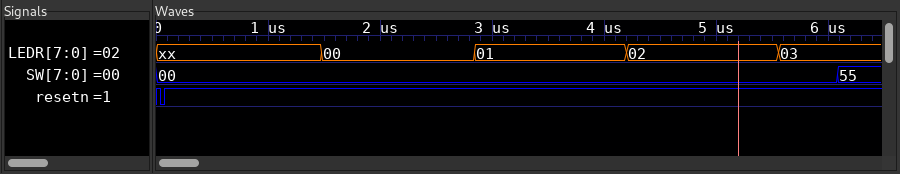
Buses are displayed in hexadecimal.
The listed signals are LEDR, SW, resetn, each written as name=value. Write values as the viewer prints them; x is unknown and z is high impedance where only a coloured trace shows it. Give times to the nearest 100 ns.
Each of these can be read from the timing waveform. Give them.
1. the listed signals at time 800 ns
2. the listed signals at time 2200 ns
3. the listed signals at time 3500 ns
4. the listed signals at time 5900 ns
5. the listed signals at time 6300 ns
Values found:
LEDR=xx, SW=00, resetn=1
LEDR=00, SW=00, resetn=1
LEDR=01, SW=00, resetn=1
LEDR=03, SW=00, resetn=1
LEDR=03, SW=55, resetn=1
